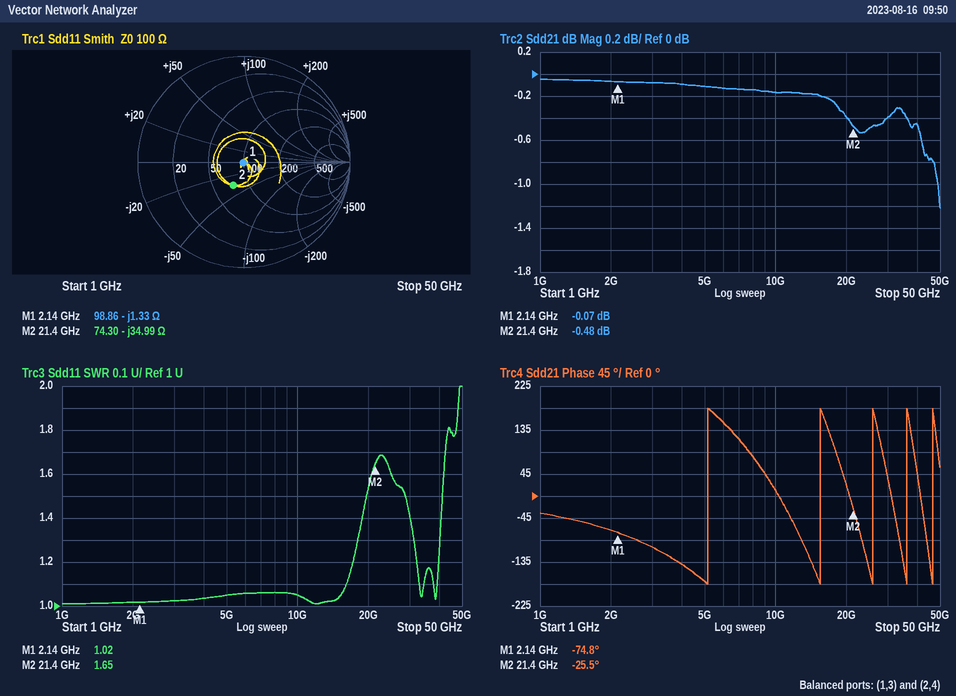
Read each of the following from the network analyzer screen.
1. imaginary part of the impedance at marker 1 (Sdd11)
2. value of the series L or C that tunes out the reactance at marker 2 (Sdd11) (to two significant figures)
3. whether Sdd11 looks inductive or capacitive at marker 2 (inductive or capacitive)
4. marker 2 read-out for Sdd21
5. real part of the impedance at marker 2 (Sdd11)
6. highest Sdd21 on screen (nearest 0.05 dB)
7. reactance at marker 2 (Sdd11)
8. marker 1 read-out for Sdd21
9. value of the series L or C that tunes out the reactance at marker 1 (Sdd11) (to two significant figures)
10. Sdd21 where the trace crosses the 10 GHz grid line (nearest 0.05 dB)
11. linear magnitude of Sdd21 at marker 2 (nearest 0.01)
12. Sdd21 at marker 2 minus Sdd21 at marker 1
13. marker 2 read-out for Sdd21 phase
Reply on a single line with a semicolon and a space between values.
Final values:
-1.33 Ω; 260 pH; capacitive; -0.48 dB; 74.30 Ω; -0.05 dB; -34.99 Ω; -0.07 dB; 99 pH; -0.15 dB; 0.95; -0.41 dB; -25.5°
